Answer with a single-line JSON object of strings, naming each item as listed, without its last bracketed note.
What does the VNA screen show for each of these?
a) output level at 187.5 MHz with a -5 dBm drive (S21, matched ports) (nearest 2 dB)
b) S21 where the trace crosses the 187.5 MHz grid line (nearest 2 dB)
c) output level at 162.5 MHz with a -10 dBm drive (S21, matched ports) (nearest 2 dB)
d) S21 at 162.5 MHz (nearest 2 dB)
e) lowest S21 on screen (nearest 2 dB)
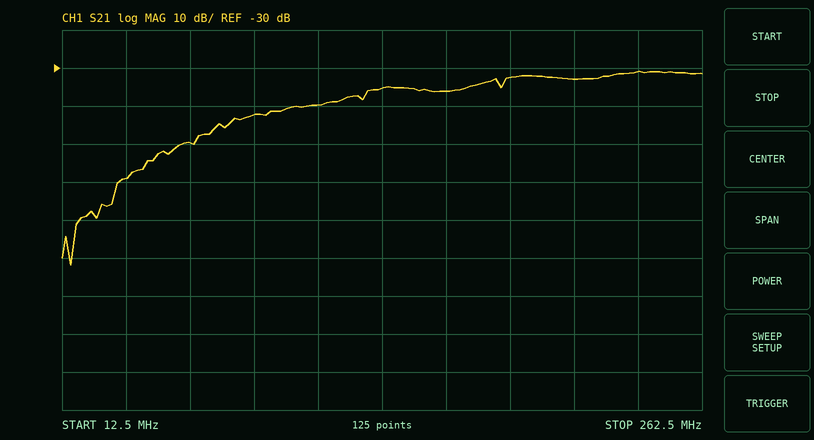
{"output level at 187.5 MHz with a -5 dBm drive (S21, matched ports)": "-38 dBm", "S21 where the trace crosses the 187.5 MHz grid line": "-32 dB", "output level at 162.5 MHz with a -10 dBm drive (S21, matched ports)": "-46 dBm", "S21 at 162.5 MHz": "-36 dB", "lowest S21 on screen": "-82 dB"}
